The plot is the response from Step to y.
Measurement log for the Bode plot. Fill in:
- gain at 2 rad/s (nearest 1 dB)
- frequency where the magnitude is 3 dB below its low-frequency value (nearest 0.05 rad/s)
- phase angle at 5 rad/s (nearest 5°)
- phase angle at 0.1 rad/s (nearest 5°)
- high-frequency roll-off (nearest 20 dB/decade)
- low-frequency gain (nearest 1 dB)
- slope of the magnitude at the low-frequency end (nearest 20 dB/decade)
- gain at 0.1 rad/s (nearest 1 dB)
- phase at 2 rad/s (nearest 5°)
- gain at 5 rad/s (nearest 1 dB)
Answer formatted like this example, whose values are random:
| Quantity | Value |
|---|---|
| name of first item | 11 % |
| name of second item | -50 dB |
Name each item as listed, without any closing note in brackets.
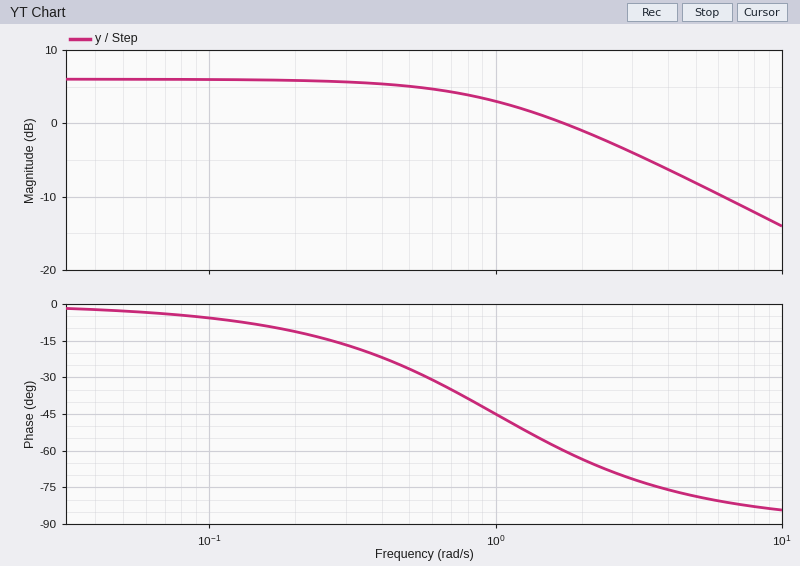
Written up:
| Quantity | Value |
|---|---|
| gain at 2 rad/s | -1 dB |
| frequency where the magnitude is 3 dB below its low-frequency value | 1.00 rad/s |
| phase angle at 5 rad/s | -80° |
| phase angle at 0.1 rad/s | -5° |
| high-frequency roll-off | -20 dB/decade |
| low-frequency gain | 6 dB |
| slope of the magnitude at the low-frequency end | 0 dB/decade |
| gain at 0.1 rad/s | 6 dB |
| phase at 2 rad/s | -65° |
| gain at 5 rad/s | -8 dB |
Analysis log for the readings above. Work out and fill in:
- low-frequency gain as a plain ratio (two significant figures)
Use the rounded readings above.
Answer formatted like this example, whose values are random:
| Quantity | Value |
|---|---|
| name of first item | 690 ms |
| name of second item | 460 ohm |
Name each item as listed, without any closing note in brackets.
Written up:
| Quantity | Value |
|---|---|
| low-frequency gain as a plain ratio | 2.0 |
